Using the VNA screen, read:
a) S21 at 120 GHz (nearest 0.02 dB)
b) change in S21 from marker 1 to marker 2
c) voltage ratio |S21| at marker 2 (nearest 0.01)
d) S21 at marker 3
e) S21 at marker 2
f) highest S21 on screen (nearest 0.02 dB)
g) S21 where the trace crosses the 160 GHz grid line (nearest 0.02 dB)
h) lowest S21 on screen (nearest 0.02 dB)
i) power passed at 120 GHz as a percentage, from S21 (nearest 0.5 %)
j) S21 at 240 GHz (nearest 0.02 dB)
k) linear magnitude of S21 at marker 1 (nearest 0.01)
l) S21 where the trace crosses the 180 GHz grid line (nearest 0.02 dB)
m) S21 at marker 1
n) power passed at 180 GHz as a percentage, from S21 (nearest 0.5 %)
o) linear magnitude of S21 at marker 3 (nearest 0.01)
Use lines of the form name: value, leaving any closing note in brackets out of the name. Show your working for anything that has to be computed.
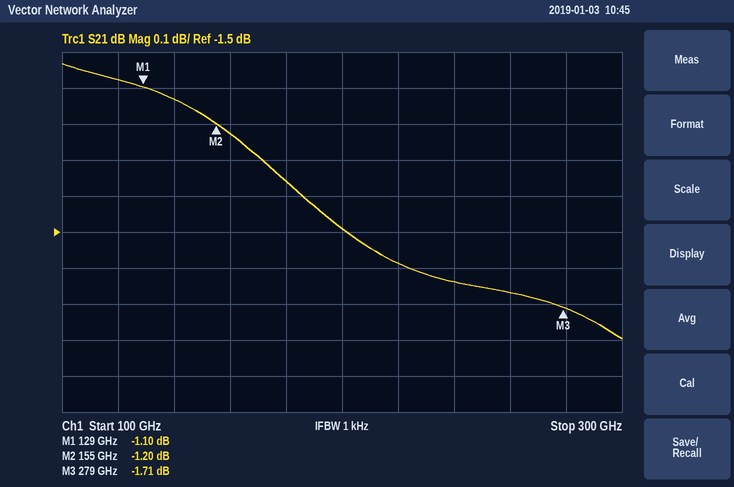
S21 at 120 GHz: -1.08 dB
change in S21 from marker 1 to marker 2: -1.2 − (-1.1) = -0.10 dB
voltage ratio |S21| at marker 2: 10^(-1.2/20) ≈ 0.87
S21 at marker 3: -1.71 dB
S21 at marker 2: -1.20 dB
highest S21 on screen: -1.04 dB
S21 where the trace crosses the 160 GHz grid line: -1.22 dB
lowest S21 on screen: -1.80 dB
power passed at 120 GHz as a percentage, from S21: 10^(-1.08/10) ≈ 78.0 %
S21 at 240 GHz: -1.64 dB
linear magnitude of S21 at marker 1: 10^(-1.1/20) ≈ 0.88
S21 where the trace crosses the 180 GHz grid line: -1.36 dB
S21 at marker 1: -1.10 dB
power passed at 180 GHz as a percentage, from S21: 10^(-1.36/10) ≈ 73.1 %, so 73.0 % to the nearest 0.5 %
linear magnitude of S21 at marker 3: 10^(-1.71/20) ≈ 0.82
